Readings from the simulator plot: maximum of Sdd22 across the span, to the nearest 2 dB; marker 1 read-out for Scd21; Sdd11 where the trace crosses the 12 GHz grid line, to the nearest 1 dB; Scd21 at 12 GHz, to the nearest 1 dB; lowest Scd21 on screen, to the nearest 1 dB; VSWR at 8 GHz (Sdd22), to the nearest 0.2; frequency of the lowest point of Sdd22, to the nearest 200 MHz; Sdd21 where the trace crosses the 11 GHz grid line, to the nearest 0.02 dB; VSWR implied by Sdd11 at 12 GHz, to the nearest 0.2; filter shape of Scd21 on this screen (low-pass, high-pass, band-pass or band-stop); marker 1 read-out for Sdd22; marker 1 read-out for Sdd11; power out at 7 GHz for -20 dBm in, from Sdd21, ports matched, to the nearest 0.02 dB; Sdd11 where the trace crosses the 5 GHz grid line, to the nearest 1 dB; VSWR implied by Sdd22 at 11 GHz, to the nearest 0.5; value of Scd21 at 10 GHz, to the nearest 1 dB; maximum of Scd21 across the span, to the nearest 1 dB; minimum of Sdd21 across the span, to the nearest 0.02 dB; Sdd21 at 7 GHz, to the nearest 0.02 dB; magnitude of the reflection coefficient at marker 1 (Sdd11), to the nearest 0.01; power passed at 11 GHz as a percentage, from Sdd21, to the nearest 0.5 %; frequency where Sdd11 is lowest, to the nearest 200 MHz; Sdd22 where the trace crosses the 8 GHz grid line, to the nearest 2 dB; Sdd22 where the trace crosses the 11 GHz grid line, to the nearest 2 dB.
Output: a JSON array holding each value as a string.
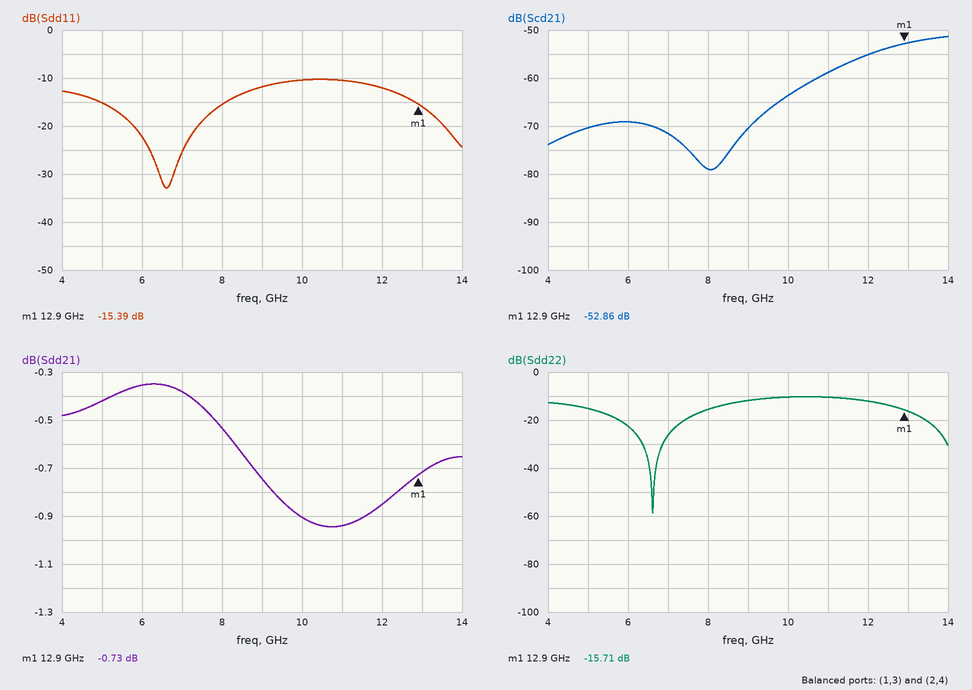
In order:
["-10 dB", "-52.86 dB", "-12 dB", "-55 dB", "-79 dB", "1.4", "6.6 GHz", "-0.94 dB", "1.6", "high-pass", "-15.71 dB", "-15.39 dB", "-20.38 dBm", "-15 dB", "2.0", "-64 dB", "-51 dB", "-0.94 dB", "-0.38 dB", "0.17", "80.5 %", "6.6 GHz", "-16 dB", "-10 dB"]
